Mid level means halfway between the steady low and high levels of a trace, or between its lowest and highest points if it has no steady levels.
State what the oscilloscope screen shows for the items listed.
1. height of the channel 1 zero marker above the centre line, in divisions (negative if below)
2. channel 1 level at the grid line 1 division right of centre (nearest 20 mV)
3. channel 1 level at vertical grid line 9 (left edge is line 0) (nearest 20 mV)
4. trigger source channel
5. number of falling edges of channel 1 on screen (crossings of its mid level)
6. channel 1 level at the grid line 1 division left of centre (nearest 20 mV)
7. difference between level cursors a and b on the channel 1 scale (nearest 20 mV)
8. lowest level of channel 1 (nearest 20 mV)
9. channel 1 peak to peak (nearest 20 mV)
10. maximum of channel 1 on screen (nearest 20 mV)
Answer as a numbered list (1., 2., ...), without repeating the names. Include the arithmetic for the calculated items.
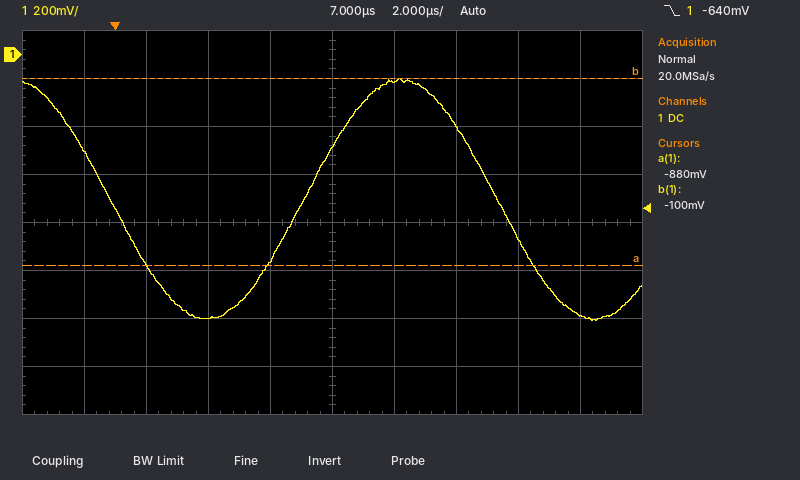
1. +3.5 div
2. -120 mV
3. -1.08 V
4. channel 1
5. 2
6. -860 mV
7. 780 mV
8. -1.10 V
9. -100 mV − (-1.10 V) = 1.00 V
10. -100 mV
